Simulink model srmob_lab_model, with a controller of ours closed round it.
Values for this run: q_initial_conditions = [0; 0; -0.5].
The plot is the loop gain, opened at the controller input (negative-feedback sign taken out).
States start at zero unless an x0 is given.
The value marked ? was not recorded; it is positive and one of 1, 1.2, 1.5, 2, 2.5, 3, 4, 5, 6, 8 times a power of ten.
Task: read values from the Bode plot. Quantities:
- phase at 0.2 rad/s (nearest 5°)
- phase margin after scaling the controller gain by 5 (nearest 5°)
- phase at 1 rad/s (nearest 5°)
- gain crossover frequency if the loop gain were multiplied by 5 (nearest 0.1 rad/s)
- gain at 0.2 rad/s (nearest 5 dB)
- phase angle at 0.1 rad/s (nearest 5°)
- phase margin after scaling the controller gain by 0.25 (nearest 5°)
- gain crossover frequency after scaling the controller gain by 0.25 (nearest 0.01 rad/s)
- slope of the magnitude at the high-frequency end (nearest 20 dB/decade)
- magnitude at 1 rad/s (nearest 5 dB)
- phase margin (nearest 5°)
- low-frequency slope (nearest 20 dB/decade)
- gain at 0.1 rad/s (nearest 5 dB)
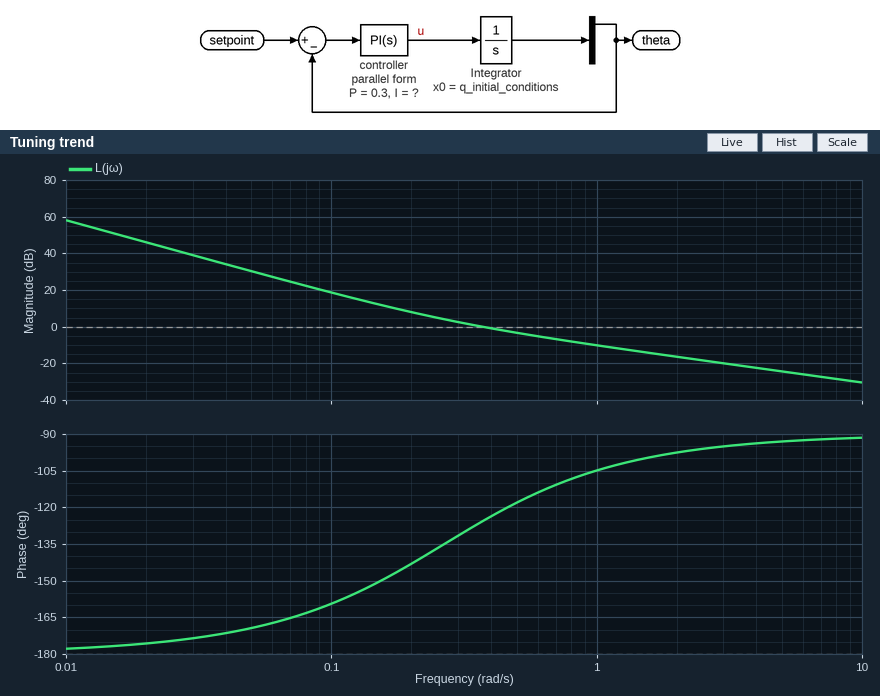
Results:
-145°
80°
-105°
1.5 rad/s
10 dB
-160°
30°
0.15 rad/s
-20 dB/decade
-10 dB
55°
-40 dB/decade
20 dB
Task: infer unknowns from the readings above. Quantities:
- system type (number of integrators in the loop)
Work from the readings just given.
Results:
2
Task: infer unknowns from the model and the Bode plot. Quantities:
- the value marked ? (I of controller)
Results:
0.08
